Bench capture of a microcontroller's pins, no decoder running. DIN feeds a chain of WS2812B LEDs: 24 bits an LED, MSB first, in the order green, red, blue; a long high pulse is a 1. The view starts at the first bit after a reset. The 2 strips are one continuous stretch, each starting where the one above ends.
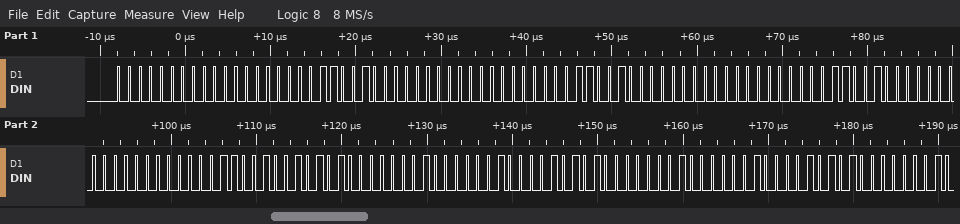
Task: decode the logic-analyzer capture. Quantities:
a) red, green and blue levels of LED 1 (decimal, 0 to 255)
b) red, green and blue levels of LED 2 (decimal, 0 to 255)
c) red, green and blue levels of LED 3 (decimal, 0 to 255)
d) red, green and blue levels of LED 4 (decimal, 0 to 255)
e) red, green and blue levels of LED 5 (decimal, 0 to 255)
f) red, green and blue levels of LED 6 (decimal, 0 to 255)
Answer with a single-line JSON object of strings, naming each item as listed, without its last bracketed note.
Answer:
{"red, green and blue levels of LED 1": "0, 0, 25", "red, green and blue levels of LED 2": "0, 0, 25", "red, green and blue levels of LED 3": "0, 0, 25", "red, green and blue levels of LED 4": "0, 0, 25", "red, green and blue levels of LED 5": "2, 42, 4", "red, green and blue levels of LED 6": "2, 42, 4"}
